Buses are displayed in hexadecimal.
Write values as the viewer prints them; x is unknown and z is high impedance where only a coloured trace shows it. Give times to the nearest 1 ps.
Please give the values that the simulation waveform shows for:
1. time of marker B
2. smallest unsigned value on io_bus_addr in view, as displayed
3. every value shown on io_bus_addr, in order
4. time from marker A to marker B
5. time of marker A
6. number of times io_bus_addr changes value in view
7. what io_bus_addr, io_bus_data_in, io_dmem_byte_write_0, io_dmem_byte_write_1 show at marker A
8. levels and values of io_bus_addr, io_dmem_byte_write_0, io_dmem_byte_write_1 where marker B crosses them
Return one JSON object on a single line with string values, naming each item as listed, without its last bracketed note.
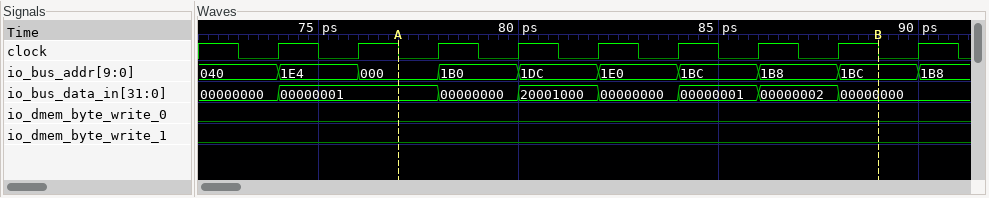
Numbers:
{"time of marker B": "89 ps", "smallest unsigned value on io_bus_addr in view, as displayed": "000", "every value shown on io_bus_addr, in order": "040, 1E4, 000, 1B0, 1DC, 1E0, 1BC, 1B8, 1BC, 1B8", "time from marker A to marker B": "12 ps", "time of marker A": "77 ps", "number of times io_bus_addr changes value in view": "9", "what io_bus_addr, io_bus_data_in, io_dmem_byte_write_0, io_dmem_byte_write_1 show at marker A": "io_bus_addr=000, io_bus_data_in=00000001, io_dmem_byte_write_0=0, io_dmem_byte_write_1=0", "levels and values of io_bus_addr, io_dmem_byte_write_0, io_dmem_byte_write_1 where marker B crosses them": "io_bus_addr=1BC, io_dmem_byte_write_0=0, io_dmem_byte_write_1=0"}
